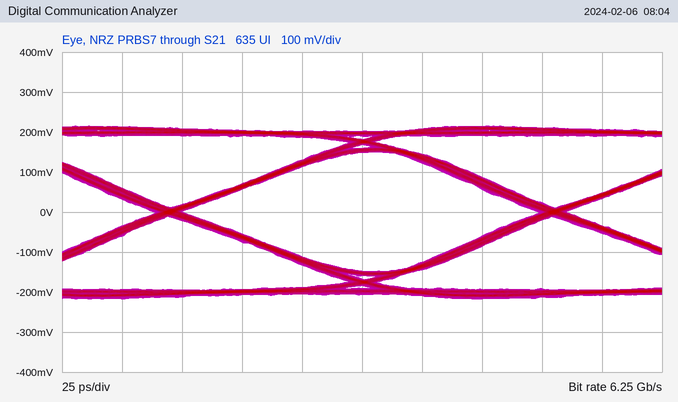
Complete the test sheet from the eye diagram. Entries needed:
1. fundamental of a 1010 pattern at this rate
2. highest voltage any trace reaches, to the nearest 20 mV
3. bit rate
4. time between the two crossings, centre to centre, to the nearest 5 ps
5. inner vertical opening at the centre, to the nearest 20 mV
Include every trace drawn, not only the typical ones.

3.125 GHz
220 mV
6.25 Gb/s
160 ps
300 mV
